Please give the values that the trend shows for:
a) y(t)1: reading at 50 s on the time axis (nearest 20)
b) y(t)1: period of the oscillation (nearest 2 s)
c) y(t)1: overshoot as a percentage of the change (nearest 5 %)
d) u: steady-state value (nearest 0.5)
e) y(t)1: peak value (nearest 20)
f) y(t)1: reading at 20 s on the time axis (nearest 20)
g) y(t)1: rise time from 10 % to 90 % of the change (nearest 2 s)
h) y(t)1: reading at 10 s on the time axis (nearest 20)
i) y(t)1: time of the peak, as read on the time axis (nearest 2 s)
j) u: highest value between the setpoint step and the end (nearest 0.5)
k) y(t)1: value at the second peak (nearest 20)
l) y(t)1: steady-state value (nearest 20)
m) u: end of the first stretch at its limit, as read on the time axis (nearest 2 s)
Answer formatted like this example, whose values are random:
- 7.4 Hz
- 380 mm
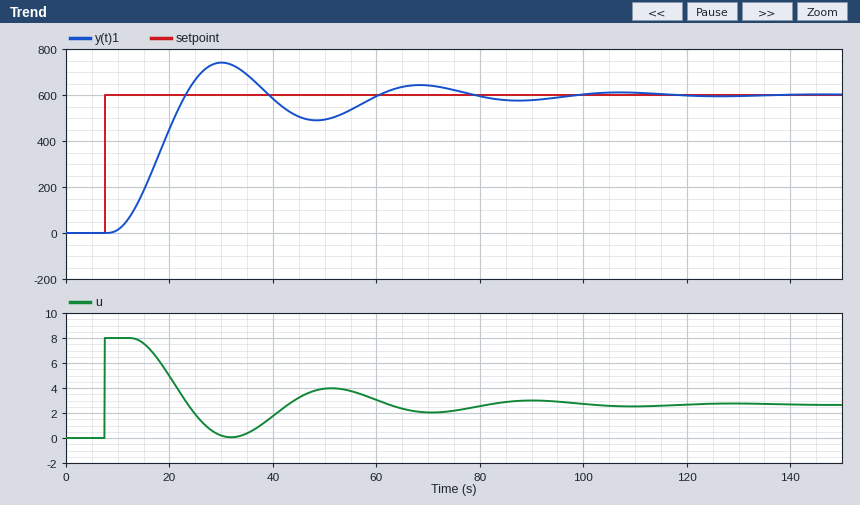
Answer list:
- 500
- 38 s
- 25 %
- 2.5
- 740
- 460
- 10 s
- 20
- 30 s
- 8.0
- 640
- 600
- 14 s
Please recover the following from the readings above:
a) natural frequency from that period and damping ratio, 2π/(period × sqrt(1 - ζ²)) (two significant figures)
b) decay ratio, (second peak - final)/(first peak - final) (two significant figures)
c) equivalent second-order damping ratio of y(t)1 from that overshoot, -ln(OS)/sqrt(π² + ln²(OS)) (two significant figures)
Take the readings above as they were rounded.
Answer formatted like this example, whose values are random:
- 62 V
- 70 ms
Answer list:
- 0.18 rad/s
- 0.29
- 0.40
